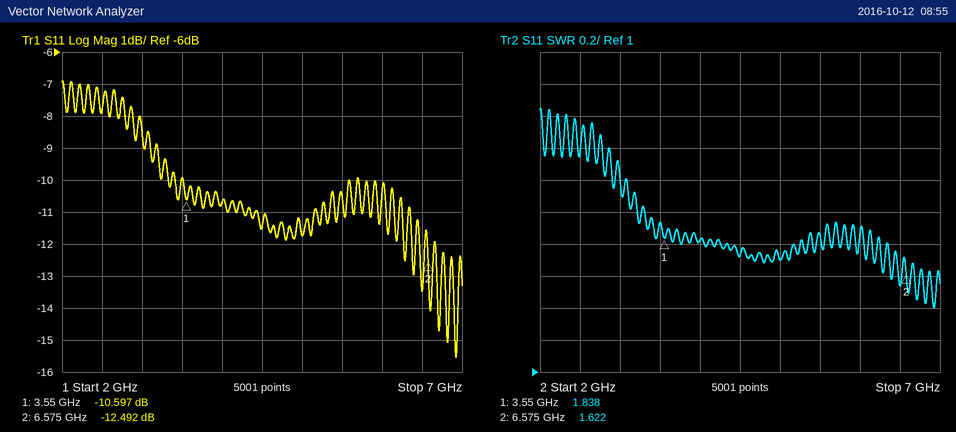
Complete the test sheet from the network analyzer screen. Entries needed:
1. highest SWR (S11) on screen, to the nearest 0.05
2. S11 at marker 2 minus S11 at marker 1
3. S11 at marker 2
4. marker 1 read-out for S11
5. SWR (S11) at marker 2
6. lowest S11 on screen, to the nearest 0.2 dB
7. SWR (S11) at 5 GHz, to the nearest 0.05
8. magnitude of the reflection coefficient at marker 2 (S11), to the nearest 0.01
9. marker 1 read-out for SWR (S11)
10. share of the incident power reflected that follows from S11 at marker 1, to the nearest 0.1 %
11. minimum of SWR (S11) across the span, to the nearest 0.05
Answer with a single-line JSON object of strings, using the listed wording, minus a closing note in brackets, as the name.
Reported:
{"highest SWR (S11) on screen, to the nearest 0.05": "2.65", "S11 at marker 2 minus S11 at marker 1": "-1.895 dB", "S11 at marker 2": "-12.492 dB", "marker 1 read-out for S11": "-10.597 dB", "SWR (S11) at marker 2": "1.622", "lowest S11 on screen, to the nearest 0.2 dB": "-15.6 dB", "SWR (S11) at 5 GHz, to the nearest 0.05": "1.70", "magnitude of the reflection coefficient at marker 2 (S11), to the nearest 0.01": "0.24", "marker 1 read-out for SWR": "1.838", "share of the incident power reflected that follows from S11 at marker 1, to the nearest 0.1 %": "8.7 %", "minimum of SWR (S11) across the span, to the nearest 0.05": "1.40"}
